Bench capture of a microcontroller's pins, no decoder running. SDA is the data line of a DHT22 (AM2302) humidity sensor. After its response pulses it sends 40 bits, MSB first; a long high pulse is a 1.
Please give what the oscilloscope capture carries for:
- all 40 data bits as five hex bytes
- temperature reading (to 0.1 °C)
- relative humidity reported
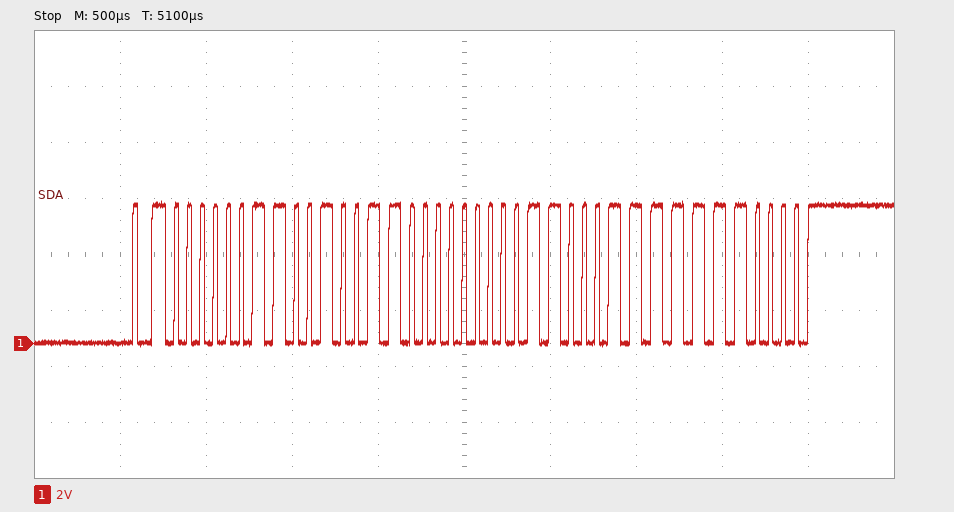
03 26 00 C7 F0
19.9 °C
80.6 %
